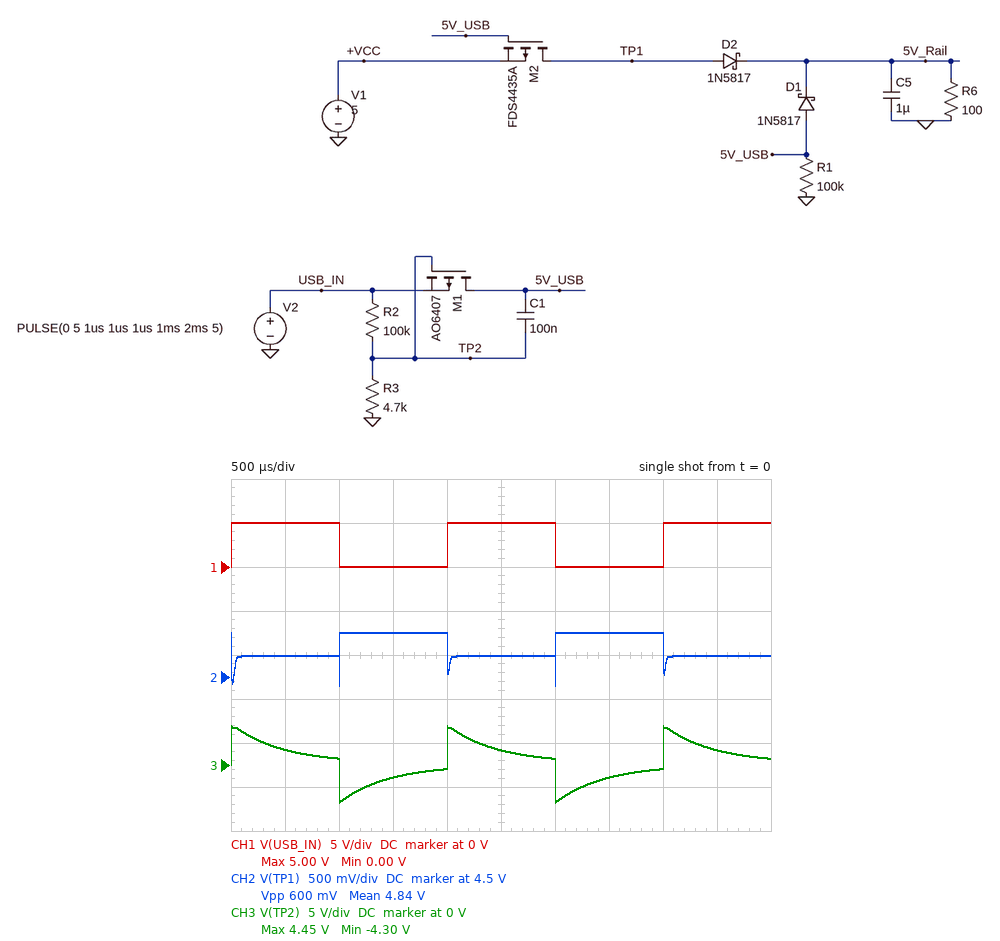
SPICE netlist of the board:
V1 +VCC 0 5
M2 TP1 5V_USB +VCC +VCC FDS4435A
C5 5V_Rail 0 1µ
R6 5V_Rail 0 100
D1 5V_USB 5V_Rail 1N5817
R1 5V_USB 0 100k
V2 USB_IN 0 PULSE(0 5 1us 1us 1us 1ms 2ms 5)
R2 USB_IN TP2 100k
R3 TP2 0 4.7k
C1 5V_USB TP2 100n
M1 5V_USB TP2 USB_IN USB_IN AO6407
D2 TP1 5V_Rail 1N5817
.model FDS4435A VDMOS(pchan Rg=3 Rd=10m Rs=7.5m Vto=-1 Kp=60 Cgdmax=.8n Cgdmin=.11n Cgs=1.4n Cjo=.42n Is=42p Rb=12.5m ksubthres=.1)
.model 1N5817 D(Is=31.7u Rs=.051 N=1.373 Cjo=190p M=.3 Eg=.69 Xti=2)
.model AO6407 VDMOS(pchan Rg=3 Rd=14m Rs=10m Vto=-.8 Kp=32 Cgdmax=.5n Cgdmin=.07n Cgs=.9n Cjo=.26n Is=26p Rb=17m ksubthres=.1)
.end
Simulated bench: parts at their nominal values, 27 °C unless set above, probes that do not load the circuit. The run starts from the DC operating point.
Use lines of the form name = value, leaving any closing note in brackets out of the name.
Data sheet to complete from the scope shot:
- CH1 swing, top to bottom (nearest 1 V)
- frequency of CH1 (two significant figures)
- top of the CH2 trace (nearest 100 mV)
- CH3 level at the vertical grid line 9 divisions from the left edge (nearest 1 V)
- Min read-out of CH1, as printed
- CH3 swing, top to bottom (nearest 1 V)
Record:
CH1 swing, top to bottom = 5 V
frequency of CH1 = 500 Hz
top of the CH2 trace = 5.0 V
CH3 level at the vertical grid line 9 divisions from the left edge = 2 V
Min read-out of CH1, as printed = 0.00 V
CH3 swing, top to bottom = 9 V
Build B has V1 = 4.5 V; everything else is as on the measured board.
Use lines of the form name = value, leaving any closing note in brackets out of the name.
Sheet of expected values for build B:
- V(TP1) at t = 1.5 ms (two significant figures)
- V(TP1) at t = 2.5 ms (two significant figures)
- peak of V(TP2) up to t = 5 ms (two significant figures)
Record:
V(TP1) at t = 1.5 ms = 4.5 V
V(TP1) at t = 2.5 ms = 4.7 V
peak of V(TP2) up to t = 5 ms = 4.2 V
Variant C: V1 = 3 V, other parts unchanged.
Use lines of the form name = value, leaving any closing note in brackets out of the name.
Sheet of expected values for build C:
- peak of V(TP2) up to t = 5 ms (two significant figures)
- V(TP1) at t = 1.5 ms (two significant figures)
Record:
peak of V(TP2) up to t = 5 ms = 4.2 V
V(TP1) at t = 1.5 ms = 3.0 V
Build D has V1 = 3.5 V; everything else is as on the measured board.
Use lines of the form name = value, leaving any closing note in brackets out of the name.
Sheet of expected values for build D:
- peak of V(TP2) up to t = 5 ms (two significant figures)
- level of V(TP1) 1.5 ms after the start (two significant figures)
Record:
peak of V(TP2) up to t = 5 ms = 4.2 V
level of V(TP1) 1.5 ms after the start = 3.5 V
